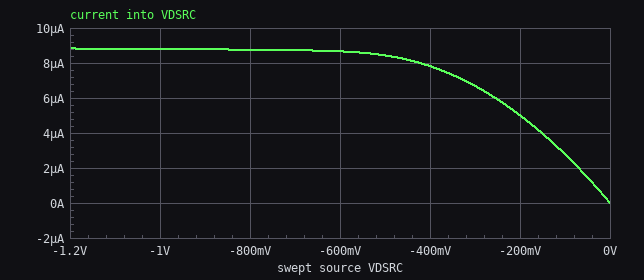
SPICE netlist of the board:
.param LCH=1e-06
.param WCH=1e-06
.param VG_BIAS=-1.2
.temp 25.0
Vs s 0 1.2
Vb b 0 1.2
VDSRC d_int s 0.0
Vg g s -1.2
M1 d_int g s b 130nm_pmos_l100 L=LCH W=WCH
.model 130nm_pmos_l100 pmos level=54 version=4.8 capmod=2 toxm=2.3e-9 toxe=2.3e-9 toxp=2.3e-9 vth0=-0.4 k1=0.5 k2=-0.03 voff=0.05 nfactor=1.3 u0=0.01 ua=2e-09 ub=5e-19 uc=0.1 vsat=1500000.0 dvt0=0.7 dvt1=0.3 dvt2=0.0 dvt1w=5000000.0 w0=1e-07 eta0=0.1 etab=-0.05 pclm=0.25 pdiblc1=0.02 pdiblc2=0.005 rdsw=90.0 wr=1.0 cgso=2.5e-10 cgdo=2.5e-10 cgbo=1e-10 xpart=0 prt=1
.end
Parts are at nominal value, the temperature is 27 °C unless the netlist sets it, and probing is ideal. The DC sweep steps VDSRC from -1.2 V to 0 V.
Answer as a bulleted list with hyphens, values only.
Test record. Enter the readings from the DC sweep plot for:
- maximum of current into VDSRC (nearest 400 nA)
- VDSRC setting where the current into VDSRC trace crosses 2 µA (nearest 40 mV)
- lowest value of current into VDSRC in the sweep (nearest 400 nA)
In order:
- 8.8 µA
- -80 mV
- 0 A
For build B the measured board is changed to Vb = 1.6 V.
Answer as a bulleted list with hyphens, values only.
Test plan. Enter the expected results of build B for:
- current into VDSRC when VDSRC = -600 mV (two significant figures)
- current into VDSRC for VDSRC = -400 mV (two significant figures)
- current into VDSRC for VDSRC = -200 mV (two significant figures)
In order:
- 190 µA
- 170 µA
- 110 µA
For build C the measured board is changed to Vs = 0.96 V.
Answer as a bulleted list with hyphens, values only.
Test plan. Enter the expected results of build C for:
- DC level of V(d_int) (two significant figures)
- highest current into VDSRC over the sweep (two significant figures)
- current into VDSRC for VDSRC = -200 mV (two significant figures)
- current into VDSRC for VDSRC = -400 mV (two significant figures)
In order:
- 960 mV
- 210 µA
- 120 µA
- 190 µA
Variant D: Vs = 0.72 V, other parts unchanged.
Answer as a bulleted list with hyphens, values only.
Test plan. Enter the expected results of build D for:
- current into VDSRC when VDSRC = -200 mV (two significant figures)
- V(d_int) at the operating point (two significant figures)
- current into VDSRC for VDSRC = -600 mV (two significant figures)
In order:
- 110 µA
- 720 mV
- 180 µA
